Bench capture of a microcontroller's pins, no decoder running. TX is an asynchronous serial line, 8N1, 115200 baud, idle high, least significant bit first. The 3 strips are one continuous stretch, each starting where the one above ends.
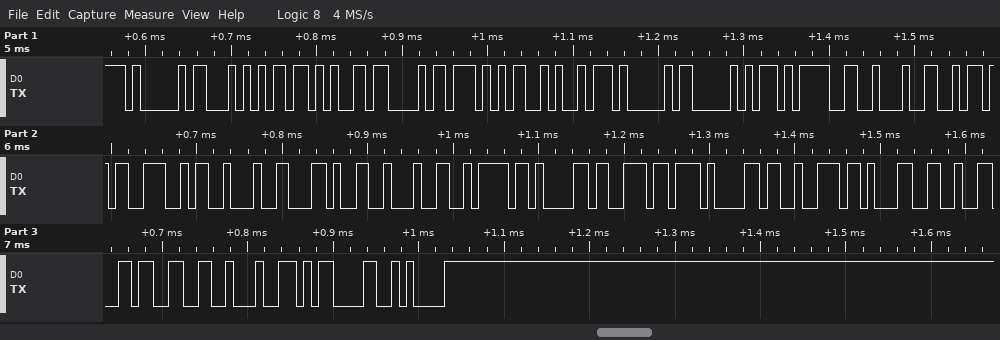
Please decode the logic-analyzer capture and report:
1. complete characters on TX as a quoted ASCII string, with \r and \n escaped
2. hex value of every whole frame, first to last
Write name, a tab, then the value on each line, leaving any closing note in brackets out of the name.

complete characters on TX as a quoted ASCII string, with \r and \n escaped	"AT+CWJAP=\"ZN\",\"zanar123\"\r\n"
hex value of every whole frame, first to last	41 54 2B 43 57 4A 41 50 3D 22 5A 4E 22 2C 22 7A 61 6E 61 72 31 32 33 22 0D 0A
